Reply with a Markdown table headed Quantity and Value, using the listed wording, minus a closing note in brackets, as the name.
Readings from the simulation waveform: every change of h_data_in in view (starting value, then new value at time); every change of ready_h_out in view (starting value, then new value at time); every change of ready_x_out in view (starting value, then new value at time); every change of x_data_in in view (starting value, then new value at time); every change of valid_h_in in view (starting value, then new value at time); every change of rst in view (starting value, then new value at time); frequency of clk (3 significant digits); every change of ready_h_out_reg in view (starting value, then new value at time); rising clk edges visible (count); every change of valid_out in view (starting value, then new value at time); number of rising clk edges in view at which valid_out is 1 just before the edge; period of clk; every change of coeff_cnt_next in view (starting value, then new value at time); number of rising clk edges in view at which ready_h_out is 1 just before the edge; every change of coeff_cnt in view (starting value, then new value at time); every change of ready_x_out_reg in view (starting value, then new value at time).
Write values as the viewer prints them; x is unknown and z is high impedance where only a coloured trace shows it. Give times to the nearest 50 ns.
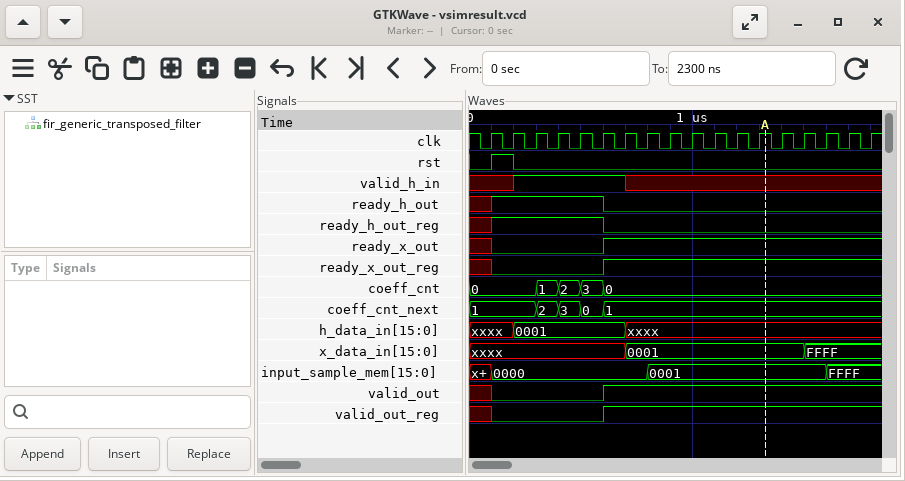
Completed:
| Quantity | Value |
|---|---|
| every change of h_data_in in view | xxxx, 0001 at 200 ns, xxxx at 700 ns |
| every change of ready_h_out in view | x, 1 at 100 ns, 0 at 600 ns |
| every change of ready_x_out in view | x, 0 at 100 ns, 1 at 600 ns |
| every change of x_data_in in view | xxxx, 0001 at 700 ns, FFFF at 1500 ns |
| every change of valid_h_in in view | x, 1 at 200 ns, x at 700 ns |
| every change of rst in view | 0, 1 at 100 ns, 0 at 200 ns |
| frequency of clk | 10.0 MHz |
| every change of ready_h_out_reg in view | x, 1 at 100 ns, 0 at 600 ns |
| rising clk edges visible | 18 |
| every change of valid_out in view | x, 0 at 100 ns, 1 at 600 ns |
| number of rising clk edges in view at which valid_out is 1 just before the edge | 12 |
| period of clk | 100 ns |
| every change of coeff_cnt_next in view | 1, 2 at 300 ns, 3 at 400 ns, 0 at 500 ns, 1 at 600 ns |
| number of rising clk edges in view at which ready_h_out is 1 just before the edge | 5 |
| every change of coeff_cnt in view | 0, 1 at 300 ns, 2 at 400 ns, 3 at 500 ns, 0 at 600 ns |
| every change of ready_x_out_reg in view | x, 0 at 100 ns, 1 at 600 ns |
